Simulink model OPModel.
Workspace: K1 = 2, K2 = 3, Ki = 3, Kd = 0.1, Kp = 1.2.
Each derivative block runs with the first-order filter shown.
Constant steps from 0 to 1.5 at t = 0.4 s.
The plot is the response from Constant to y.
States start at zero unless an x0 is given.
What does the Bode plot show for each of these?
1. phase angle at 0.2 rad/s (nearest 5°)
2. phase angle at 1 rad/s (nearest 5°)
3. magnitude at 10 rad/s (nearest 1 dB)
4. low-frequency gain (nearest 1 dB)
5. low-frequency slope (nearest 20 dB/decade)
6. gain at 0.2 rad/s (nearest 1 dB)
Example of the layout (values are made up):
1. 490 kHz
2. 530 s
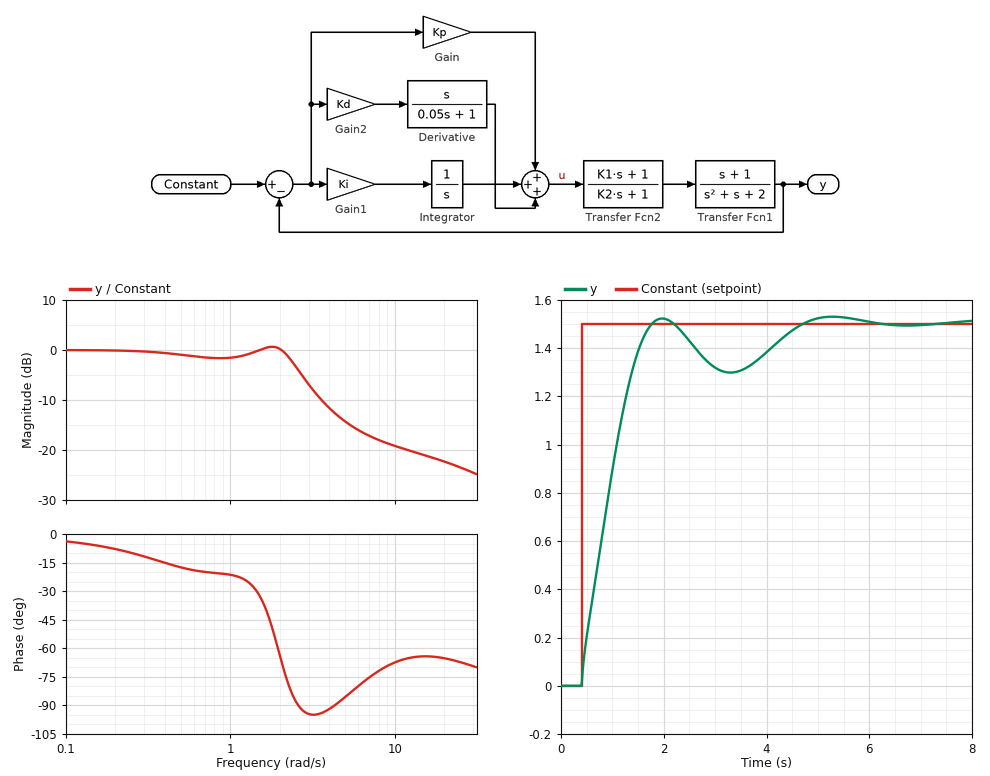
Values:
1. -10°
2. -20°
3. -19 dB
4. 0 dB
5. 0 dB/decade
6. 0 dB
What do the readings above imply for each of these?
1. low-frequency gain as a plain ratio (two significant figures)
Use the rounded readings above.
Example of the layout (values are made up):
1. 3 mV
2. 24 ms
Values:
1. 1.0
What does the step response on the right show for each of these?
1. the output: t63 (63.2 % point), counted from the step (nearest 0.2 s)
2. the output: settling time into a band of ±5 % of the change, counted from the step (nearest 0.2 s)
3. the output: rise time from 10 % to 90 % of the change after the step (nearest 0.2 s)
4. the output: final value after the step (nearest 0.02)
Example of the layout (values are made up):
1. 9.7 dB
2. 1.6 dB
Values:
1. 0.6 s
2. 3.8 s
3. 1.0 s
4. 1.50
